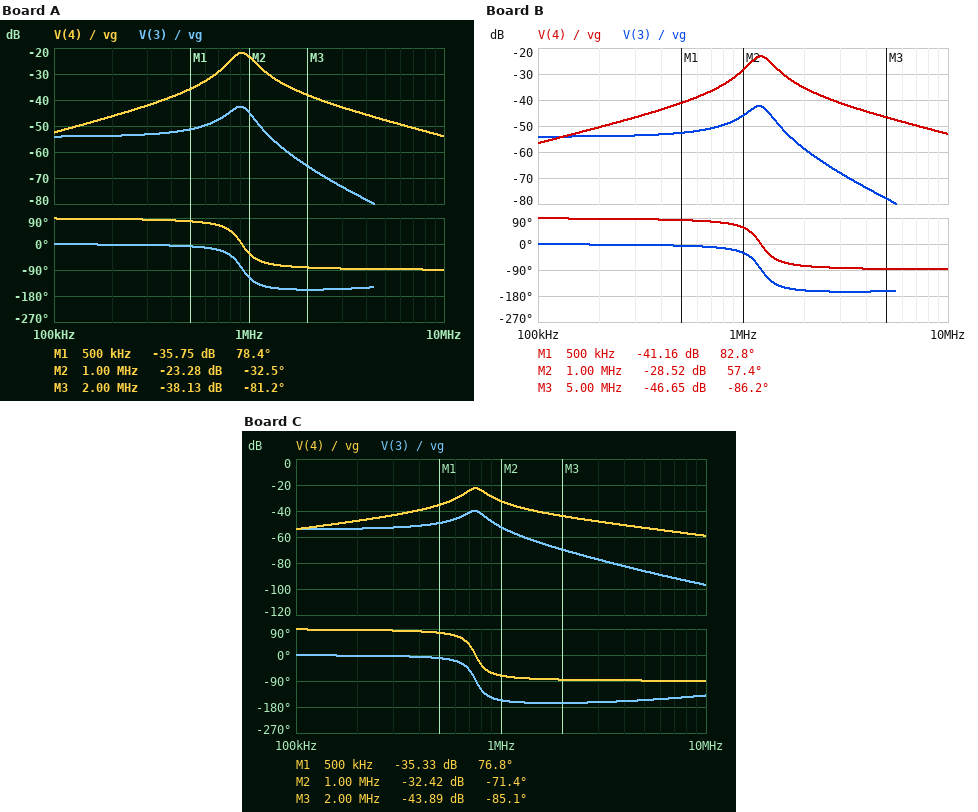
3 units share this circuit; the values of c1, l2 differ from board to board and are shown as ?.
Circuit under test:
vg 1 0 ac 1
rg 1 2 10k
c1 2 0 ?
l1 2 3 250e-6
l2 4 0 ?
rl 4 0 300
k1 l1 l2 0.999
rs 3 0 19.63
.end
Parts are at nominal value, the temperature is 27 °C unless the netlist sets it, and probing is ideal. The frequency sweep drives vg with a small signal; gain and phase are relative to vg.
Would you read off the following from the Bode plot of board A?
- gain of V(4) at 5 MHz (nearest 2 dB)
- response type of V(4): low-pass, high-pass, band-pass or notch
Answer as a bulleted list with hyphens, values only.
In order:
- -48 dB
- band-pass
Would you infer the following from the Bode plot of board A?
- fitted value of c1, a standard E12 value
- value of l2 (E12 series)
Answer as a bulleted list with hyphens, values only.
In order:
- 120 pF
- 5.6 µH
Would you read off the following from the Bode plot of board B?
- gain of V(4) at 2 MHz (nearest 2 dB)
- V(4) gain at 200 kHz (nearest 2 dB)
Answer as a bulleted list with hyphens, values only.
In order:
- -36 dB
- -50 dB
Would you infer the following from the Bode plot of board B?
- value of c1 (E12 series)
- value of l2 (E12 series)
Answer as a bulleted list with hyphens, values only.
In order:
- 68 pF
- 2.2 µH
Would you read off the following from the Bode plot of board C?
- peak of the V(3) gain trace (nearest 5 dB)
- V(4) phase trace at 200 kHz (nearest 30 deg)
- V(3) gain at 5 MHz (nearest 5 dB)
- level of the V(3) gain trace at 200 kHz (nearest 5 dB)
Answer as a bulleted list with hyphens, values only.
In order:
- -40 dB
- 90 deg
- -85 dB
- -55 dB
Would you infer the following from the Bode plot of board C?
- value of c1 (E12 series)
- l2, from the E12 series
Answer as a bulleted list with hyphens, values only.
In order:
- 180 pF
- 3.9 µH
